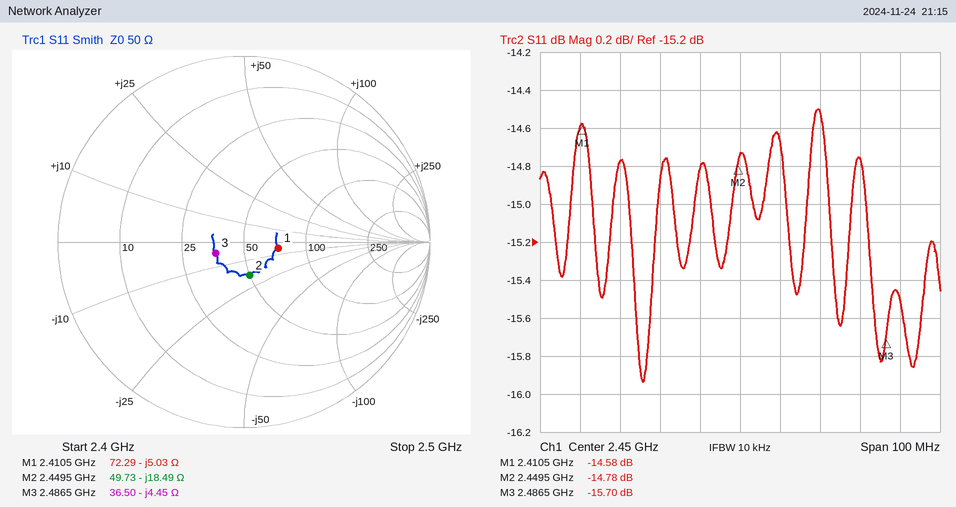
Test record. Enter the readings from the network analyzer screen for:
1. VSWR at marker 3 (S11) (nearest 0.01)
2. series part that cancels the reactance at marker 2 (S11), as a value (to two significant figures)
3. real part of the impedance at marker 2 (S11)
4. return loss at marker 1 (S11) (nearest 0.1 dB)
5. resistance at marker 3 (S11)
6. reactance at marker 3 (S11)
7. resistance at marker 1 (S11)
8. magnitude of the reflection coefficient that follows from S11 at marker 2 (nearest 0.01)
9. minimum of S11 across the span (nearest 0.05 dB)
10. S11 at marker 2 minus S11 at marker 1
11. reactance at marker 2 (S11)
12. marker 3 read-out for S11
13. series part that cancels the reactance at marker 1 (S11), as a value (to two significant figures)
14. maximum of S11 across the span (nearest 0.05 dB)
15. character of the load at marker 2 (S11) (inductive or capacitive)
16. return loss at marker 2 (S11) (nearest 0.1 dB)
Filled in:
1.39
1.2 nH
49.73 Ω
14.6 dB
36.50 Ω
-4.45 Ω
72.29 Ω
0.18
-15.95 dB
-0.20 dB
-18.49 Ω
-15.70 dB
330 pH
-14.50 dB
capacitive
14.8 dB
